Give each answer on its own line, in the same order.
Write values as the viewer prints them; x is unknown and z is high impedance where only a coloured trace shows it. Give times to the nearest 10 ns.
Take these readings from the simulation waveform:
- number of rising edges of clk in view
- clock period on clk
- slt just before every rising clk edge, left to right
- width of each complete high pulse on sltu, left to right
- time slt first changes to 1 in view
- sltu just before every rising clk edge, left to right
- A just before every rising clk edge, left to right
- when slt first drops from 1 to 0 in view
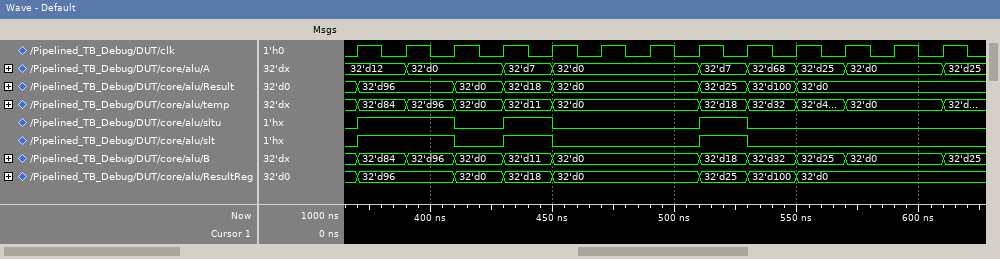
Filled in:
13
20 ns
0 1 1 0 1 0 0 0 1 0 0 0 0
40 ns, 20 ns, 20 ns
370 ns
0 1 1 0 1 0 0 0 1 0 0 0 0
32'd12, 32'd12, 32'd0, 32'd0, 32'd7, 32'd0, 32'd0, 32'd0, 32'd7, 32'd68, 32'd25, 32'd0, 32'd0
410 ns
